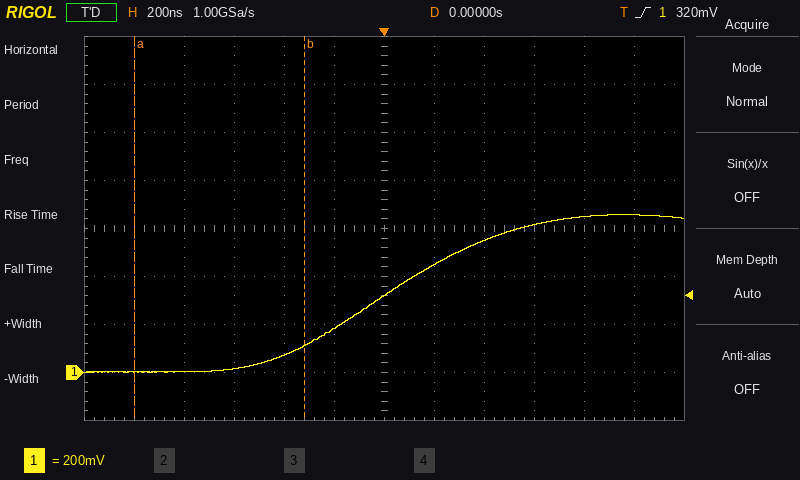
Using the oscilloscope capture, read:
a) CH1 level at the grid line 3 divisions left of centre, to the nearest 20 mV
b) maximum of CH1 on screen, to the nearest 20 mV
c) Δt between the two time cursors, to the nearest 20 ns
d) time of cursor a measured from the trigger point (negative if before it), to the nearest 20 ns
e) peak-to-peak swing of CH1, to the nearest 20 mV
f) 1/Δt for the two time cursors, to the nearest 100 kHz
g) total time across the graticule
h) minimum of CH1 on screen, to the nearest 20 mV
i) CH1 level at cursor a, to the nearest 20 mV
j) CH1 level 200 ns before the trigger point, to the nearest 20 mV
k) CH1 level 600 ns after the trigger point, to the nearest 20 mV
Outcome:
20 mV
660 mV
680 ns
-1.00 µs
660 mV
1.5 MHz
2.4 µs
0 mV
0 mV
180 mV
620 mV
